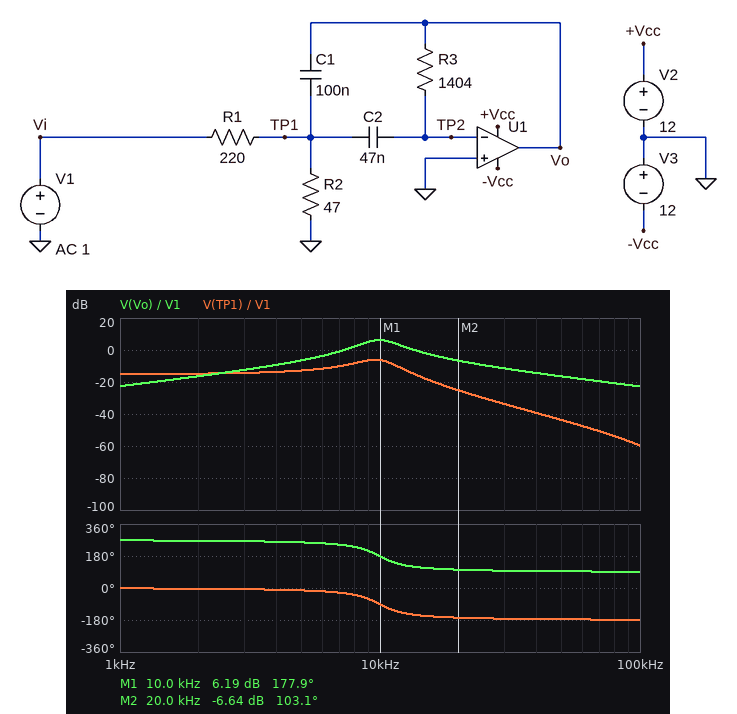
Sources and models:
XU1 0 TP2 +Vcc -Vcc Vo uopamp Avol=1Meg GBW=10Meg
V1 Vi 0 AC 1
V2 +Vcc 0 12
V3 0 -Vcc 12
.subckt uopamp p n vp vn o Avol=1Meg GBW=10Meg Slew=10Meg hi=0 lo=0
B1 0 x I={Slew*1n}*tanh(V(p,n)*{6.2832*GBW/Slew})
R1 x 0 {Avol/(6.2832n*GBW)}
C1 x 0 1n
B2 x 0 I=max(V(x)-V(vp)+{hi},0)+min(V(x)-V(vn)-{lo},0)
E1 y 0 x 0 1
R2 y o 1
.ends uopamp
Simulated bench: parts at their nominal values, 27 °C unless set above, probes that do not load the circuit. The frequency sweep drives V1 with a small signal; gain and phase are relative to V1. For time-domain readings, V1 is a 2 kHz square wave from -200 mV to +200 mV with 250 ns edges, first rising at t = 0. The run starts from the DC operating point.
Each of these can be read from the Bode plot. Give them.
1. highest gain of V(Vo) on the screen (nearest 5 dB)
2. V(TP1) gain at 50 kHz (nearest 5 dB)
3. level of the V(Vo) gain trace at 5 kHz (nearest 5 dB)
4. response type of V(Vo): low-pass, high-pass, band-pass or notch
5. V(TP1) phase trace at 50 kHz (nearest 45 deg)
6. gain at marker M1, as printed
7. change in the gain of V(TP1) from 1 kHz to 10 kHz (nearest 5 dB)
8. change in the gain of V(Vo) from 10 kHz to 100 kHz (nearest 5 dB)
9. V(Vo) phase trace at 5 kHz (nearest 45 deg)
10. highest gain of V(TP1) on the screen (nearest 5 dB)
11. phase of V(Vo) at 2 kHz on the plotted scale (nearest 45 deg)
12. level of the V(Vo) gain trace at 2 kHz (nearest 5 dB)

5 dB
-45 dB
-5 dB
band-pass
-180 deg
6.19 dB
10 dB
-30 dB
270 deg
-5 dB
270 deg
-15 dB
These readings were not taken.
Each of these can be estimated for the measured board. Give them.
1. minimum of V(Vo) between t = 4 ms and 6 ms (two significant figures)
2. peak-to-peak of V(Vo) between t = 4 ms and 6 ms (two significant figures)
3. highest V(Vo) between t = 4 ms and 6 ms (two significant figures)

-240 mV
480 mV
240 mV
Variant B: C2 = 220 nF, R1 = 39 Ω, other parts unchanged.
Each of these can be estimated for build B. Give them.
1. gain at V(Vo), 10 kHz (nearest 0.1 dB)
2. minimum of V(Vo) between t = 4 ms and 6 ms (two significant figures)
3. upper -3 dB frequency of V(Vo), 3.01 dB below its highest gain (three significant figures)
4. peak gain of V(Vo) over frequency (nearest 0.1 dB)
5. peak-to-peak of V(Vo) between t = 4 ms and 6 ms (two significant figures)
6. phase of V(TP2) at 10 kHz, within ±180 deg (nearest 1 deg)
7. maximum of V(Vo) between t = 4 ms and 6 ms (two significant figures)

16.0 dB
-3.0 V
7.05 kHz
27.9 dB
6.0 V
15 deg
3.0 V
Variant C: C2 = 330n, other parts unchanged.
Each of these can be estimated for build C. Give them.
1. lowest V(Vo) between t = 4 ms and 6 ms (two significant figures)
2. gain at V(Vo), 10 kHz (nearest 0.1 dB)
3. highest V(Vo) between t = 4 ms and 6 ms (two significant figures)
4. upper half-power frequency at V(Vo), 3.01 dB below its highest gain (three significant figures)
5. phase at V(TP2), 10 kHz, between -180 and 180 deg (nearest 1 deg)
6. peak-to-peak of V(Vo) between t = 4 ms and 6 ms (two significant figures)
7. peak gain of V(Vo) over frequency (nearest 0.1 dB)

-470 mV
-1.7 dB
470 mV
4.56 kHz
10 deg
930 mV
13.8 dB
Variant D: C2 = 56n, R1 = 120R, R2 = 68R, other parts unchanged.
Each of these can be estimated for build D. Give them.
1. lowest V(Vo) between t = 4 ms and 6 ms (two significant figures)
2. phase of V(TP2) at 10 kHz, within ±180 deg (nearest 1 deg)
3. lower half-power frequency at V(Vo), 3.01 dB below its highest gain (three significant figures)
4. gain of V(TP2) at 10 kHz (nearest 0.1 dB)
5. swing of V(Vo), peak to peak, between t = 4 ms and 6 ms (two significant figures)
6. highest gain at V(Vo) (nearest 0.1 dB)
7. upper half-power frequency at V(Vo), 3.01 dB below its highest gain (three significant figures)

-440 mV
51 deg
7.17 kHz
-49.8 dB
880 mV
12.5 dB
10.3 kHz
